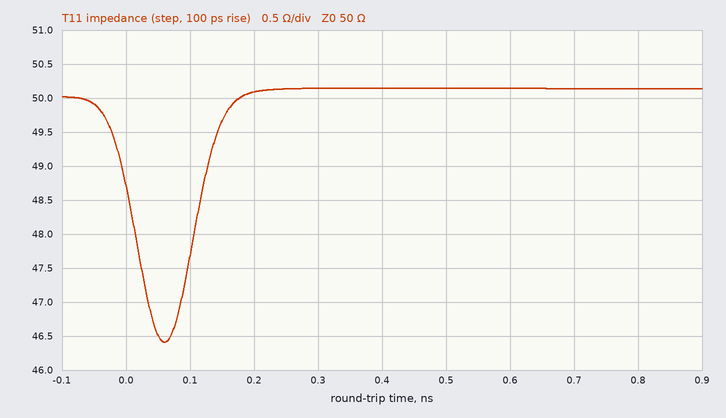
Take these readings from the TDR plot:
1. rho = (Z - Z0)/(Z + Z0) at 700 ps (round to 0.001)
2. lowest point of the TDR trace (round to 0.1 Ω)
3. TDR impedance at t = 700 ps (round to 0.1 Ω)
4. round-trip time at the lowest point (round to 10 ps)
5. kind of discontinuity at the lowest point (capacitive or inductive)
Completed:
+0.001
46.4 Ω
50.1 Ω
60 ps
capacitive
